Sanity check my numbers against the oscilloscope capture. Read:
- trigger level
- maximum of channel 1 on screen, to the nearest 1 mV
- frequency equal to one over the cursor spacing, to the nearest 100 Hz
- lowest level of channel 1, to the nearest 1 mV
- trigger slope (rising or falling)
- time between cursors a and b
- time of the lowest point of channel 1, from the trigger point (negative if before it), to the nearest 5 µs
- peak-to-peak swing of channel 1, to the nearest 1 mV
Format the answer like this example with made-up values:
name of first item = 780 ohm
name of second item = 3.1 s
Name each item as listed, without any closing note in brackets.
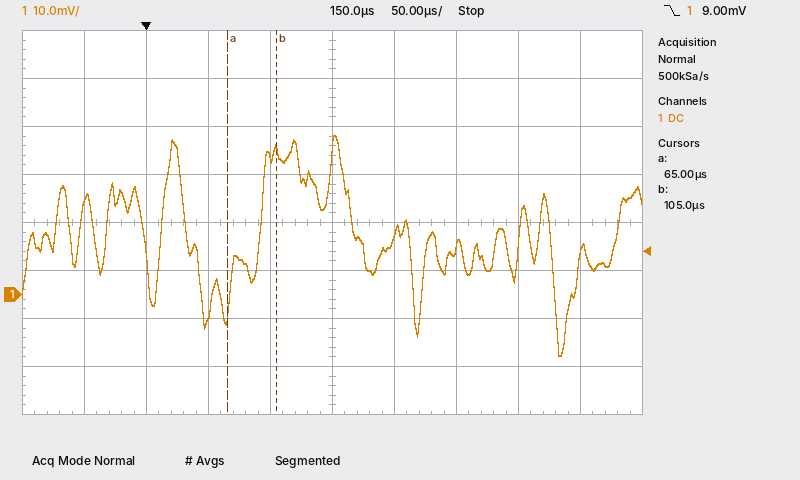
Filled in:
trigger level = 9.00 mV
maximum of channel 1 on screen, to the nearest 1 mV = 33 mV
frequency equal to one over the cursor spacing, to the nearest 100 Hz = 25.0 kHz
lowest level of channel 1, to the nearest 1 mV = -13 mV
trigger slope = falling
time between cursors a and b = 40 µs
time of the lowest point of channel 1, from the trigger point (negative if before it), to the nearest 5 µs = +335 µs
peak-to-peak swing of channel 1, to the nearest 1 mV = 46 mV
